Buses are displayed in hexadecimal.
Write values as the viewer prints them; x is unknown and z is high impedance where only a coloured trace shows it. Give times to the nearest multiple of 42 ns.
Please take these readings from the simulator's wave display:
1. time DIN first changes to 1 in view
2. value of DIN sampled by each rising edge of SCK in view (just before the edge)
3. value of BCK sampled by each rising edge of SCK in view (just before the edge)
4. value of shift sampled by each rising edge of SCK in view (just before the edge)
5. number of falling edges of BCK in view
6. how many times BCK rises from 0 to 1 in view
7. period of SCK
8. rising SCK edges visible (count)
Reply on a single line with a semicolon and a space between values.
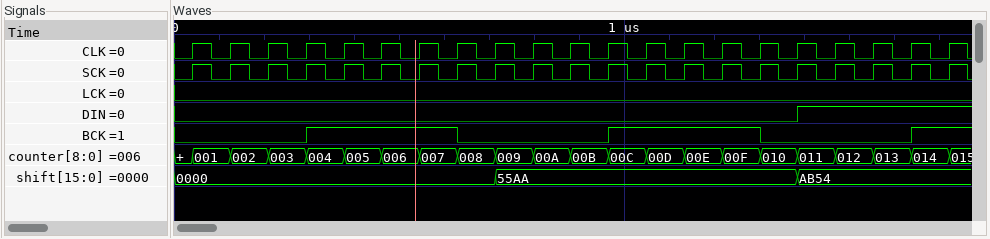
1386 ns; 0 0 0 0 0 0 0 0 0 0 0 0 0 0 0 0 0 1 1 1 1; 0 0 0 0 1 1 1 1 0 0 0 0 1 1 1 1 0 0 0 0 1; 0000, 0000, 0000, 0000, 0000, 0000, 0000, 0000, 0000, 55AA, 55AA, 55AA, 55AA, 55AA, 55AA, 55AA, 55AA, AB54, AB54, AB54, AB54; 2; 3; 84 ns; 21
